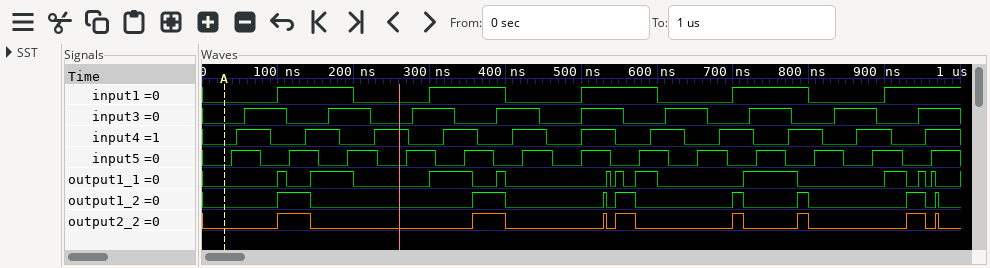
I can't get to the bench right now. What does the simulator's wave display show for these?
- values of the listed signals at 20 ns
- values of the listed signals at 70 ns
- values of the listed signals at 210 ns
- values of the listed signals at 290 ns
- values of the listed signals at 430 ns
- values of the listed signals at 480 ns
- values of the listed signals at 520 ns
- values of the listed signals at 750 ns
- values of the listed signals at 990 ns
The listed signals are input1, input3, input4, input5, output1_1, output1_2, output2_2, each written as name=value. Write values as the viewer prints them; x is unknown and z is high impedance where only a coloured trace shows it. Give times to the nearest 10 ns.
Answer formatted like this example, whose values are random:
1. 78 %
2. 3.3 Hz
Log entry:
1. input1=0, input3=0, input4=0, input5=0, output1_1=0, output1_2=0, output2_2=0
2. input1=0, input3=1, input4=1, input5=1, output1_1=0, output1_2=0, output2_2=0
3. input1=0, input3=1, input4=0, input5=1, output1_1=0, output1_2=0, output2_2=0
4. input1=0, input3=1, input4=0, input5=1, output1_1=0, output1_2=0, output2_2=0
5. input1=0, input3=1, input4=1, input5=1, output1_1=0, output1_2=0, output2_2=0
6. input1=0, input3=0, input4=0, input5=0, output1_1=0, output1_2=0, output2_2=0
7. input1=1, input3=1, input4=1, input5=1, output1_1=0, output1_2=0, output2_2=0
8. input1=1, input3=1, input4=0, input5=1, output1_1=1, output1_2=0, output2_2=0
9. input1=1, input3=1, input4=1, input5=1, output1_1=0, output1_2=0, output2_2=0
